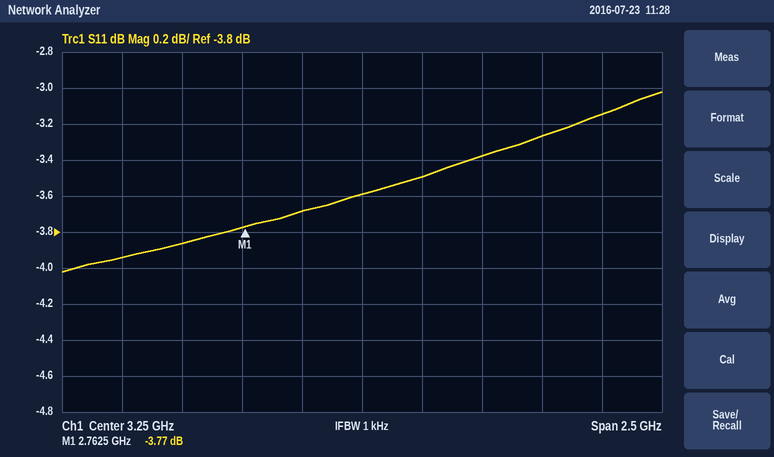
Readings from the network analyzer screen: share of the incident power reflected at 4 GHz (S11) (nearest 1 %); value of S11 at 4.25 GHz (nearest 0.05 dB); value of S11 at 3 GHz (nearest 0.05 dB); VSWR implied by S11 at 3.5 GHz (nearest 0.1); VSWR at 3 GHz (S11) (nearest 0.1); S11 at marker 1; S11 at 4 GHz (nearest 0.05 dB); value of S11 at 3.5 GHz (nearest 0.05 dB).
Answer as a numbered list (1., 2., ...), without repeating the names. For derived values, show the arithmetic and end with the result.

1. 10^(-3.25/10) ≈ 47 %
2. -3.15 dB
3. -3.70 dB
4. |Γ| = 10^(-3.5/20) = 0.6683; VSWR = (1 + 0.6683)/(1 − 0.6683) ≈ 5.0
5. |Γ| = 10^(-3.7/20) = 0.6531; VSWR = (1 + 0.6531)/(1 − 0.6531) ≈ 4.8
6. -3.77 dB
7. -3.25 dB
8. -3.50 dB
